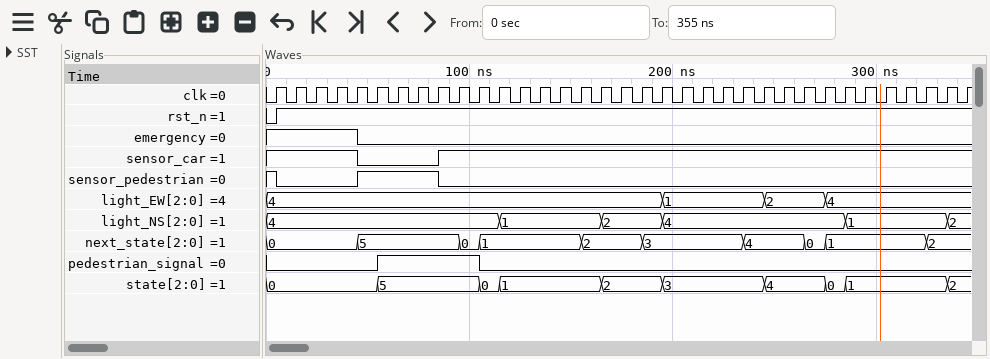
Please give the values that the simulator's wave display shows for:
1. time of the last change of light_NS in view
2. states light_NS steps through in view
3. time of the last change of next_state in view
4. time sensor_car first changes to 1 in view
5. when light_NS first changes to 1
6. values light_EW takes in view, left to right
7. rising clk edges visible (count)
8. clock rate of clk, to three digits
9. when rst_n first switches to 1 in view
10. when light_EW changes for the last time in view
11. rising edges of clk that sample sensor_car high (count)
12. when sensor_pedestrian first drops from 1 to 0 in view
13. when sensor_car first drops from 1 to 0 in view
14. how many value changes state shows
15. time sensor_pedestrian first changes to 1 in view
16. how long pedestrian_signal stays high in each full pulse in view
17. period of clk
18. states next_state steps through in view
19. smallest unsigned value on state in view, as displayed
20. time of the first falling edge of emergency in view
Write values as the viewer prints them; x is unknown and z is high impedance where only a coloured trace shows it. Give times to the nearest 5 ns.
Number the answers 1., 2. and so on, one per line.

1. 335 ns
2. 4, 1, 2, 4, 1, 2
3. 325 ns
4. 85 ns
5. 115 ns
6. 4, 1, 2, 4
7. 35
8. 100 MHz
9. 5 ns
10. 275 ns
11. 31
12. 5 ns
13. 45 ns
14. 9
15. 45 ns
16. 50 ns
17. 10 ns
18. 0, 5, 0, 1, 2, 3, 4, 0, 1, 2
19. 0
20. 45 ns
